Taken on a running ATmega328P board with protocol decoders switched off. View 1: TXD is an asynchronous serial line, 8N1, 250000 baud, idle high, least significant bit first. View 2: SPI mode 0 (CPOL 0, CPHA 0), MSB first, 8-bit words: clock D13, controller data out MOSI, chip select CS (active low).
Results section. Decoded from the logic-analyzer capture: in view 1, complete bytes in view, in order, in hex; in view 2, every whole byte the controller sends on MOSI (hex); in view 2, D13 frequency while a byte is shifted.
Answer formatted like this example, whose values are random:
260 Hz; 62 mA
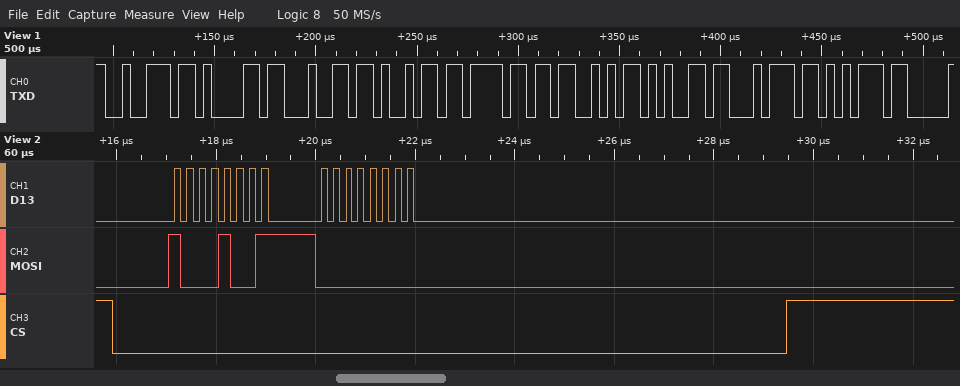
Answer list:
72 61 64 69 6F 53 65 74 75; 89 00; 4 MHz
